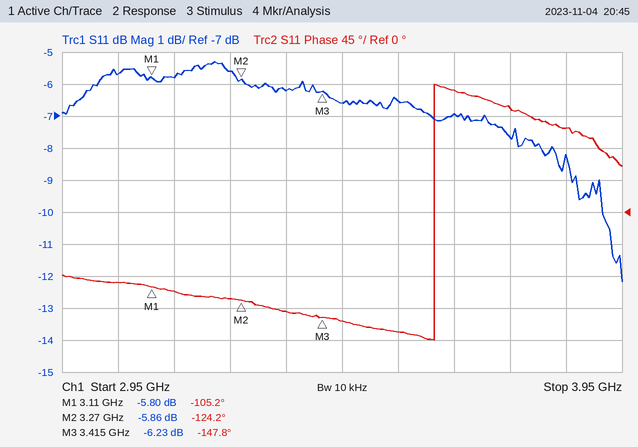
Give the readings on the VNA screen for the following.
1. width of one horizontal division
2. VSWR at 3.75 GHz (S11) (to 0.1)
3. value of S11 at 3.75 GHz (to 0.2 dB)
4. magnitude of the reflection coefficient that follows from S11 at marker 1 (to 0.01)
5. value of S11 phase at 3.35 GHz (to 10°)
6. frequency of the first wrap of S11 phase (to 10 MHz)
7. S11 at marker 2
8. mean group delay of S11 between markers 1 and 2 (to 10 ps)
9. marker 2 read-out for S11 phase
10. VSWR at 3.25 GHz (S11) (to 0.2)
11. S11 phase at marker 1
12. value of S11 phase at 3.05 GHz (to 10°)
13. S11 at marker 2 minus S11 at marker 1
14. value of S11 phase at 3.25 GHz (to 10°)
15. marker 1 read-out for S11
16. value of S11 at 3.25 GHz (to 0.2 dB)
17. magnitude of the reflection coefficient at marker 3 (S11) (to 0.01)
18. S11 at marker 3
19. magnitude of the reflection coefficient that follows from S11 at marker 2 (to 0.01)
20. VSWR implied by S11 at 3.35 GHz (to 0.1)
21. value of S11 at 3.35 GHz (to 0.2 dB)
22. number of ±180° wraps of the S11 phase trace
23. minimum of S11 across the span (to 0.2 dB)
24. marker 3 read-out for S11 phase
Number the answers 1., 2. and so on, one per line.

1. 100 MHz
2. 2.4
3. -7.6 dB
4. 0.51
5. -140°
6. 3.62 GHz
7. -5.86 dB
8. 330 ps
9. -124.2°
10. 3.2
11. -105.2°
12. -100°
13. -0.06 dB
14. -120°
15. -5.80 dB
16. -5.6 dB
17. 0.49
18. -6.23 dB
19. 0.51
20. 2.9
21. -6.2 dB
22. 1
23. -12.2 dB
24. -147.8°
